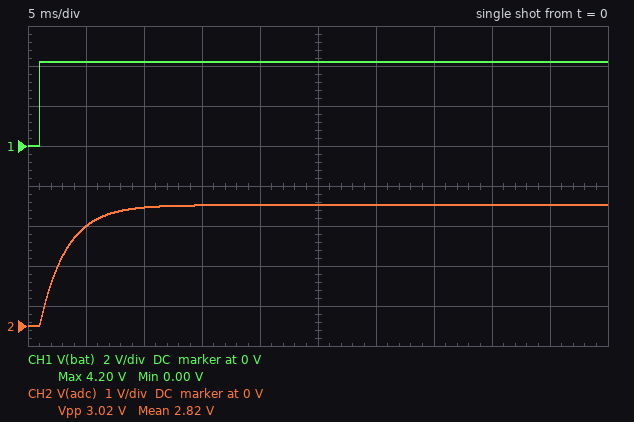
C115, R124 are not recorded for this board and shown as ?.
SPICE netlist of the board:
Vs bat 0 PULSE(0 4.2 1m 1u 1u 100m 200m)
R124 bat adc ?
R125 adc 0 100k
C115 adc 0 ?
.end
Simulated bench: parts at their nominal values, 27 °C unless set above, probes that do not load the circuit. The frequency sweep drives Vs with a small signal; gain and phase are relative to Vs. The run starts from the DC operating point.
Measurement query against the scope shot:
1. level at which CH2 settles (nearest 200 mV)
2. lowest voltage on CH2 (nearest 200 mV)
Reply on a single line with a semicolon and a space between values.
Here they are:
3.0 V; 0 V
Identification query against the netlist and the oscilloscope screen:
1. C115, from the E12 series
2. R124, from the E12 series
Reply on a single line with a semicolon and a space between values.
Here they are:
82 nF; 39 kΩ
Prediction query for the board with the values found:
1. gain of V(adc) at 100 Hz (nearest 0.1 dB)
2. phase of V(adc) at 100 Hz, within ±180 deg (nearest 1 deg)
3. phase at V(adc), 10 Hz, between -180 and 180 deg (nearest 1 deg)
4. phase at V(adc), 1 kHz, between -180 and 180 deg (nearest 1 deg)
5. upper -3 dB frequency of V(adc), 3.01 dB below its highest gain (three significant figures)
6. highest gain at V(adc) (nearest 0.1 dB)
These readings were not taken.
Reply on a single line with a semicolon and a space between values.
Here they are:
-7.8 dB; -55 deg; -8 deg; -86 deg; 69.2 Hz; -2.9 dB
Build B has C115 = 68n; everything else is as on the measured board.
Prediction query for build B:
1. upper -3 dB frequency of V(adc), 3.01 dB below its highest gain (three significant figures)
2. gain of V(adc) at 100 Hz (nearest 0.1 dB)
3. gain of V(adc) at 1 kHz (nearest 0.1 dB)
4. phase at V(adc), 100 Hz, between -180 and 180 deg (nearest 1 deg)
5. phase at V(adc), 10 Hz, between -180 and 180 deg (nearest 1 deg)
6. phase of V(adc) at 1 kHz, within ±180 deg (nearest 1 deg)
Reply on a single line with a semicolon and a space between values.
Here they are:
83.4 Hz; -6.7 dB; -24.5 dB; -50 deg; -7 deg; -85 deg
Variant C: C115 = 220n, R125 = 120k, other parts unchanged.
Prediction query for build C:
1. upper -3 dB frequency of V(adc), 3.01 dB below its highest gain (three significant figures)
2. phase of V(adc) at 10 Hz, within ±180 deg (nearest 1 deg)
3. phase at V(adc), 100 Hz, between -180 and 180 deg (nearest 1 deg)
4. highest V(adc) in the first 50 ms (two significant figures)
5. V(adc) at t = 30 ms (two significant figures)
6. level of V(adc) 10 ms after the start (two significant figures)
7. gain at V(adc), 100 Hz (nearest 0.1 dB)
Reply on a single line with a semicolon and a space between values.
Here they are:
24.6 Hz; -22 deg; -76 deg; 3.2 V; 3.1 V; 2.4 V; -14.9 dB
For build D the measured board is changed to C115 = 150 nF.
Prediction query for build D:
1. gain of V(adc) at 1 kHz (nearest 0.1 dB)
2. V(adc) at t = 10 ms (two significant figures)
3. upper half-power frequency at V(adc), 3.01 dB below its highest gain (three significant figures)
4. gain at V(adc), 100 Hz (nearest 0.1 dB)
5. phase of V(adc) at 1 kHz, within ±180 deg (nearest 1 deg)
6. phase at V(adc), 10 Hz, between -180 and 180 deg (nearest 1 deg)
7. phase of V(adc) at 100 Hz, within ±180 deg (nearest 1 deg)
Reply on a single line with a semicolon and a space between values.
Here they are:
-31.3 dB; 2.7 V; 37.8 Hz; -11.9 dB; -88 deg; -15 deg; -69 deg
